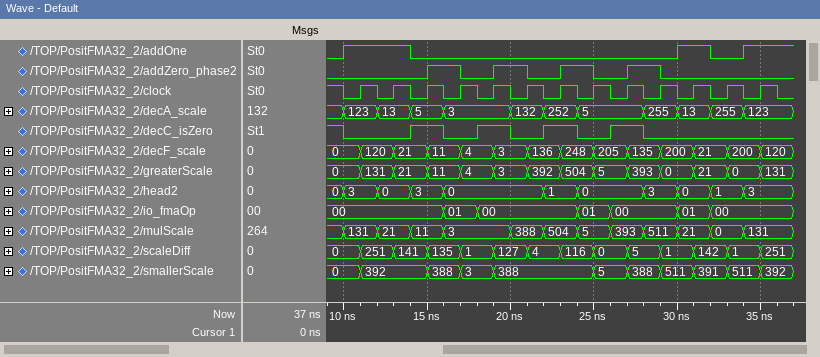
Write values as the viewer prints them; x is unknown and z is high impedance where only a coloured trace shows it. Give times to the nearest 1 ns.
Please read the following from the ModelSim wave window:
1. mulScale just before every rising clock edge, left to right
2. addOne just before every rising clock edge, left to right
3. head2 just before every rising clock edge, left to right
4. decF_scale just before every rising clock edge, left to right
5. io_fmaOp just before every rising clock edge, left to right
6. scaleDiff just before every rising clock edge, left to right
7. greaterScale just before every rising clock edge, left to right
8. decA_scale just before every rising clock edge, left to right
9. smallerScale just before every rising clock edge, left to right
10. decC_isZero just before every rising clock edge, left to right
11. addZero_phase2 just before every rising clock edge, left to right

131, 21, 11, 3, 3, 388, 504, 5, 393, 511, 21, 0, 131
1 1 0 0 0 0 0 0 0 0 1 0 1
3, 0, 3, 0, 0, 0, 1, 0, 0, 3, 0, 1, 3
0, 120, 21, 11, 4, 3, 136, 248, 205, 135, 200, 21, 200
00, 00, 00, 01, 00, 00, 00, 01, 00, 00, 01, 00, 00
0, 251, 141, 135, 1, 127, 4, 116, 0, 5, 1, 142, 1
0, 131, 21, 11, 4, 3, 392, 504, 5, 393, 0, 21, 0
123, 13, 5, 3, 3, 132, 252, 5, 5, 255, 13, 255, 123
0, 392, 392, 388, 3, 388, 388, 388, 5, 388, 511, 391, 511
0 0 1 0 1 0 1 0 1 0 0 0 0
0 0 0 1 0 1 0 1 0 1 0 0 0
